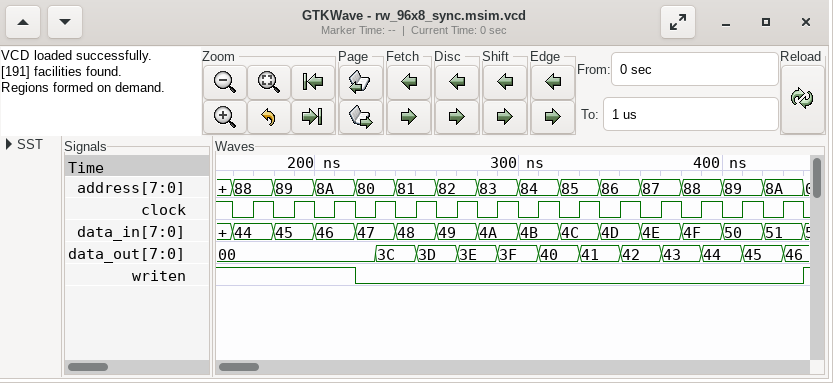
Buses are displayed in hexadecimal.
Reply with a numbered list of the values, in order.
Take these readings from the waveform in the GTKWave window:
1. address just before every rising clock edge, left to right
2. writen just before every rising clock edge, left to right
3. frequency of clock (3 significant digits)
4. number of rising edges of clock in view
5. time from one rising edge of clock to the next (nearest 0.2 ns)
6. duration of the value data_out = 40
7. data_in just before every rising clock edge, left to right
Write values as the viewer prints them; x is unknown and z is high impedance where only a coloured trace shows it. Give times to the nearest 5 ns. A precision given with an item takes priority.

1. 88, 89, 8A, 80, 81, 82, 83, 84, 85, 86, 87, 88, 89, 8A
2. 1 1 1 0 0 0 0 0 0 0 0 0 0 0
3. 50.0 MHz
4. 14
5. 20 ns
6. 20 ns
7. 44, 45, 46, 47, 48, 49, 4A, 4B, 4C, 4D, 4E, 4F, 50, 51
